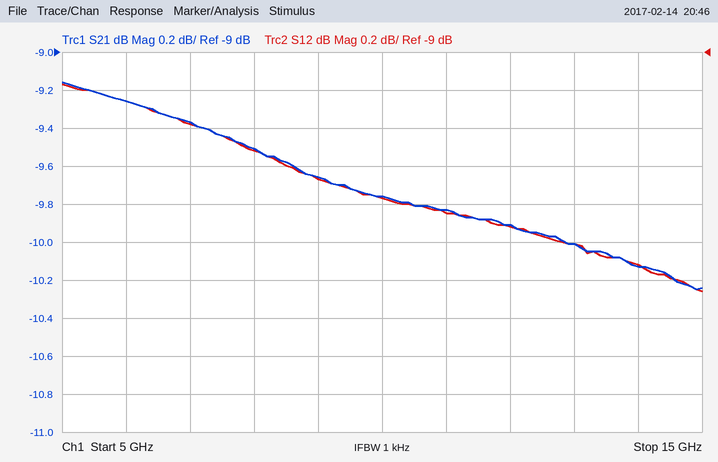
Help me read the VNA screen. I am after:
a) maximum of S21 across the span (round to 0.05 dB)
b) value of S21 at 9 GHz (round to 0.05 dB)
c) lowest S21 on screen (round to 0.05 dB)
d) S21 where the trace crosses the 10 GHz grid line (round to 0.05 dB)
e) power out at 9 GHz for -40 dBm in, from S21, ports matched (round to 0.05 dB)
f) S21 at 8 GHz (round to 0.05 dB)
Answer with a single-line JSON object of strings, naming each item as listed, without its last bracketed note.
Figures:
{"maximum of S21 across the span": "-9.15 dB", "value of S21 at 9 GHz": "-9.65 dB", "lowest S21 on screen": "-10.25 dB", "S21 where the trace crosses the 10 GHz grid line": "-9.75 dB", "power out at 9 GHz for -40 dBm in, from S21, ports matched": "-49.65 dBm", "S21 at 8 GHz": "-9.50 dB"}
